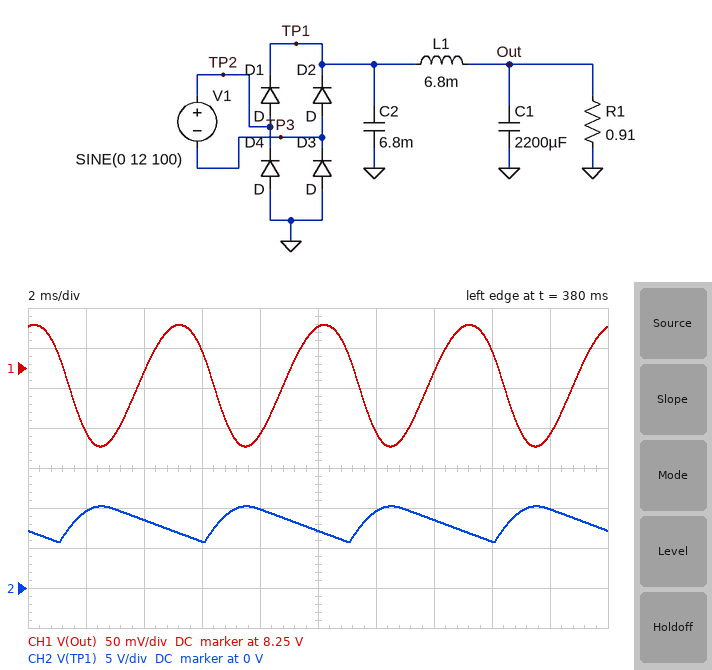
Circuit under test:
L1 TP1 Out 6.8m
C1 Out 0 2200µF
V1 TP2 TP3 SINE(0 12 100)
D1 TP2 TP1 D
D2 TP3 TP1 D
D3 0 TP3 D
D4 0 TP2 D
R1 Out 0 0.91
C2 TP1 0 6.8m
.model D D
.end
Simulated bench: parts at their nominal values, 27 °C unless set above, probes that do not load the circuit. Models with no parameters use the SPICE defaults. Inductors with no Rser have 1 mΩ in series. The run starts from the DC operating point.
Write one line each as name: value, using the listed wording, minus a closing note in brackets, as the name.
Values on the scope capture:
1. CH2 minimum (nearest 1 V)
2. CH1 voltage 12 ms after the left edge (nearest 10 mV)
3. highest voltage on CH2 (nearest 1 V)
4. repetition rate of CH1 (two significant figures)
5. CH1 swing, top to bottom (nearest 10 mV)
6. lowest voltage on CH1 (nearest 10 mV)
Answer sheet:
CH2 minimum: 6 V
CH1 voltage 12 ms after the left edge: 8.17 V
highest voltage on CH2: 10 V
repetition rate of CH1: 200 Hz
CH1 swing, top to bottom: 150 mV
lowest voltage on CH1: 8.15 V
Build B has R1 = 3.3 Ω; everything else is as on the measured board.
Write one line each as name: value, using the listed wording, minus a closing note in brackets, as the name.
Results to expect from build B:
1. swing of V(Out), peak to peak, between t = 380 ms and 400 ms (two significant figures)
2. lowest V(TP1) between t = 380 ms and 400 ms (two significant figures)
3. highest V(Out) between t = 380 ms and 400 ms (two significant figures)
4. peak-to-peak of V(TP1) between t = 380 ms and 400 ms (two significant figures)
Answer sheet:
swing of V(Out), peak to peak, between t = 380 ms and 400 ms: 57 mV
lowest V(TP1) between t = 380 ms and 400 ms: 8.6 V
highest V(Out) between t = 380 ms and 400 ms: 9.5 V
peak-to-peak of V(TP1) between t = 380 ms and 400 ms: 1.7 V
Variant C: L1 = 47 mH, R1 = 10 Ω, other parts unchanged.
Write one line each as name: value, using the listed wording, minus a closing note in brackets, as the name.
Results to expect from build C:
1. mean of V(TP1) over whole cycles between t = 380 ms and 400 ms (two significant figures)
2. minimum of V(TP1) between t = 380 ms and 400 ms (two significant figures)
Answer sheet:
mean of V(TP1) over whole cycles between t = 380 ms and 400 ms: 10 V
minimum of V(TP1) between t = 380 ms and 400 ms: 9.7 V
